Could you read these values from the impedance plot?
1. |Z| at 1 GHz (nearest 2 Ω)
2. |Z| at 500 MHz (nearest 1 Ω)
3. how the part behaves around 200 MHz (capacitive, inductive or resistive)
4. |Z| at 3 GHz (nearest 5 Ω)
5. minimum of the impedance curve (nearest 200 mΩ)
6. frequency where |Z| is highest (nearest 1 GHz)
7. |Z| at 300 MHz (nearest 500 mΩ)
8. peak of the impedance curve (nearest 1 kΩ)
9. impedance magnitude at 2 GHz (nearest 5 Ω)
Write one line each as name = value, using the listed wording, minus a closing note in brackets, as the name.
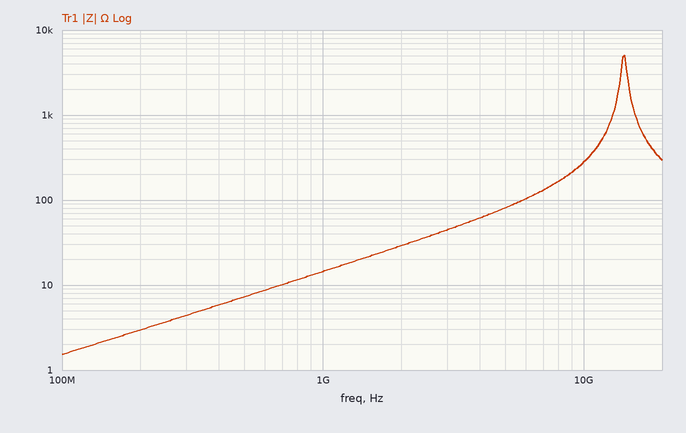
|Z| at 1 GHz = 14 Ω
|Z| at 500 MHz = 7 Ω
how the part behaves around 200 MHz = inductive
|Z| at 3 GHz = 45 Ω
minimum of the impedance curve = 1.6 Ω
frequency where |Z| is highest = 14 GHz
|Z| at 300 MHz = 4.5 Ω
peak of the impedance curve = 5 kΩ
impedance magnitude at 2 GHz = 30 Ω
